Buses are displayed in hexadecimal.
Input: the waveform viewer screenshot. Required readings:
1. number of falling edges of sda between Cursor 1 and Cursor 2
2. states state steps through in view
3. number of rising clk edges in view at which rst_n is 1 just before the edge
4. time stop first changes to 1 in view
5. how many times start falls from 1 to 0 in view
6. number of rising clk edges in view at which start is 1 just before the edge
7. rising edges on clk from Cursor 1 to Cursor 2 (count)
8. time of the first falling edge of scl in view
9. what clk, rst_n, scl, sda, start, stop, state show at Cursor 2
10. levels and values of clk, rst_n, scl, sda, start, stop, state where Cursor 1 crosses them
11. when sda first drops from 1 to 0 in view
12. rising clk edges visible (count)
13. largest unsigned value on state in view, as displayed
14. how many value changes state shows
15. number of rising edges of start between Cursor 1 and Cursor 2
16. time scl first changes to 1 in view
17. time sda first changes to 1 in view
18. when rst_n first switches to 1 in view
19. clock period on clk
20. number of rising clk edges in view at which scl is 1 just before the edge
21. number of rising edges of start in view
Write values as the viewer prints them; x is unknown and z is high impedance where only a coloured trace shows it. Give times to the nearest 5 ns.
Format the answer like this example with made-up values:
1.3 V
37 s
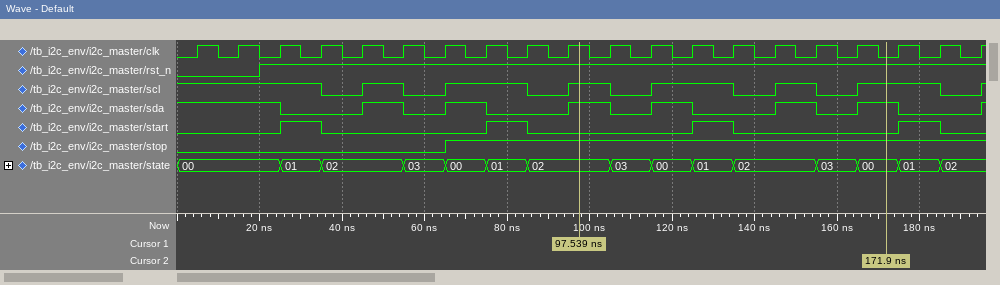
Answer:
3
00, 01, 02, 03, 00, 01, 02, 03, 00, 01, 02, 03, 00, 01, 02
18
65 ns
4
4
7
35 ns
clk=0, rst_n=1, scl=1, sda=1, start=0, stop=1, state=00
clk=1, rst_n=1, scl=1, sda=1, start=0, stop=1, state=02
25 ns
20
03
14
1
45 ns
45 ns
20 ns
10 ns
13
4
